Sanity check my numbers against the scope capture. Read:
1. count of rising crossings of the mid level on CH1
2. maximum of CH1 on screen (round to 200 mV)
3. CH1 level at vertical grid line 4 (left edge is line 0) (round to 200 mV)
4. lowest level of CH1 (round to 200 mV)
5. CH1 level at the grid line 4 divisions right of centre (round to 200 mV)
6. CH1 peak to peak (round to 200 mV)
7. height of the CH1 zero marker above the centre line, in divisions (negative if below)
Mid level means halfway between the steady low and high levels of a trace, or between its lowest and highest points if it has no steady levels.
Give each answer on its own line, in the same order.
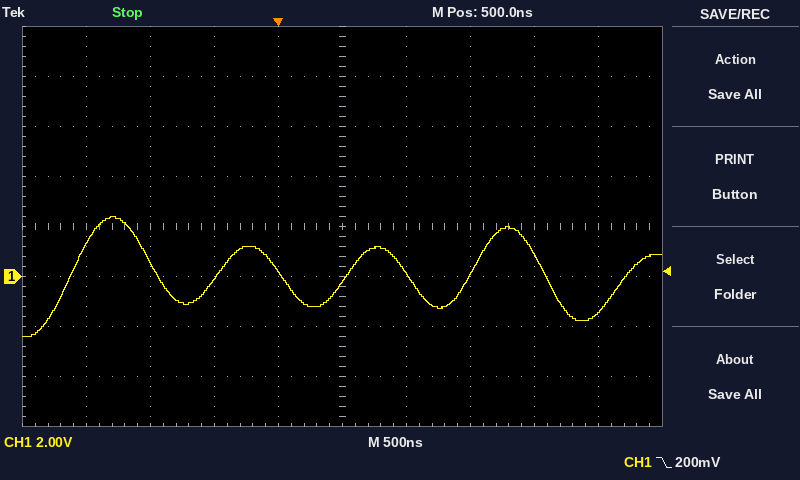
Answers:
5
2.4 V
200 mV
-2.4 V
-1.4 V
4.8 V
-1.0 div
